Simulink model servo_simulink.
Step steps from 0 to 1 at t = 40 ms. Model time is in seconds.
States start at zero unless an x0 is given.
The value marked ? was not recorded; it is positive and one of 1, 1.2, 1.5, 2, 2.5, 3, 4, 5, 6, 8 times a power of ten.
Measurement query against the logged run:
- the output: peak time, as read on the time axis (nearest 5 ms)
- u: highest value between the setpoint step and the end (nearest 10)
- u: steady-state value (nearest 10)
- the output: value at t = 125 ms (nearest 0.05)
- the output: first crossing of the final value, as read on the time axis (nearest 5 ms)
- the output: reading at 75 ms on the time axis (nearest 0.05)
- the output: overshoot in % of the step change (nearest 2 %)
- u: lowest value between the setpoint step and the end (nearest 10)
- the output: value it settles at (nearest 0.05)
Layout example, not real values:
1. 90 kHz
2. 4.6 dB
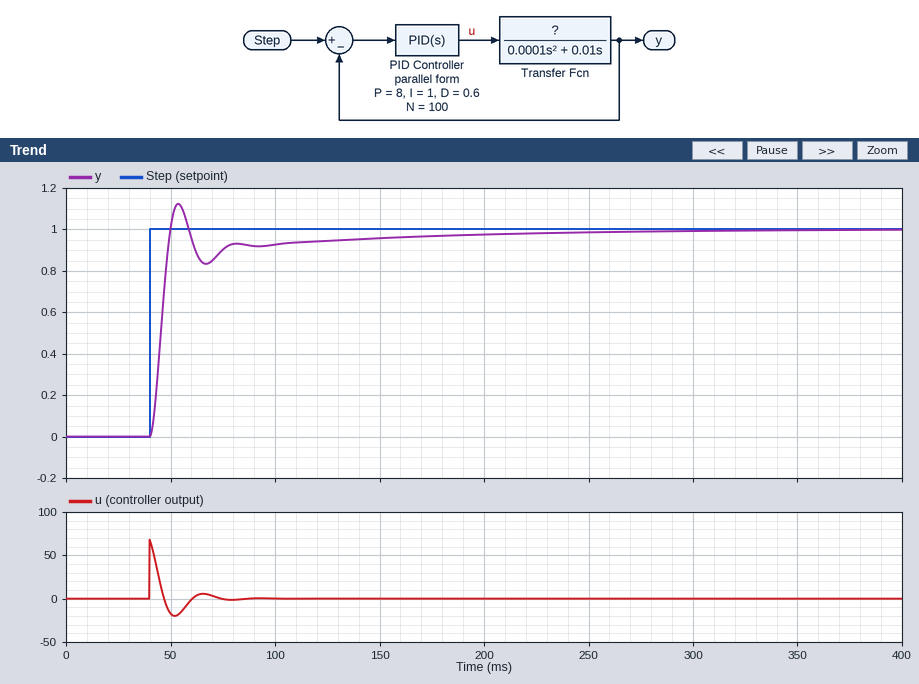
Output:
1. 55 ms
2. 70
3. 0
4. 0.95
5. 50 ms
6. 0.90
7. 12 %
8. -20
9. 1.00
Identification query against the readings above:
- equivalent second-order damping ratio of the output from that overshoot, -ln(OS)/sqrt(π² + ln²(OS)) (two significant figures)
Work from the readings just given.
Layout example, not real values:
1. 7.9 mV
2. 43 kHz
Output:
1. 0.56
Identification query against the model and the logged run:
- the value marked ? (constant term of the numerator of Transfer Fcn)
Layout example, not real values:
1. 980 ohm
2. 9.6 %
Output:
1. 0.08
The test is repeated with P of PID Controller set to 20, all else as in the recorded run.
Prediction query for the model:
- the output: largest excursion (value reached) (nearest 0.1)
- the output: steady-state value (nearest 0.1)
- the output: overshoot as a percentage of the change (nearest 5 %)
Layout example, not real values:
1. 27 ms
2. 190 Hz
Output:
1. 1.2
2. 1.0
3. 25 %
